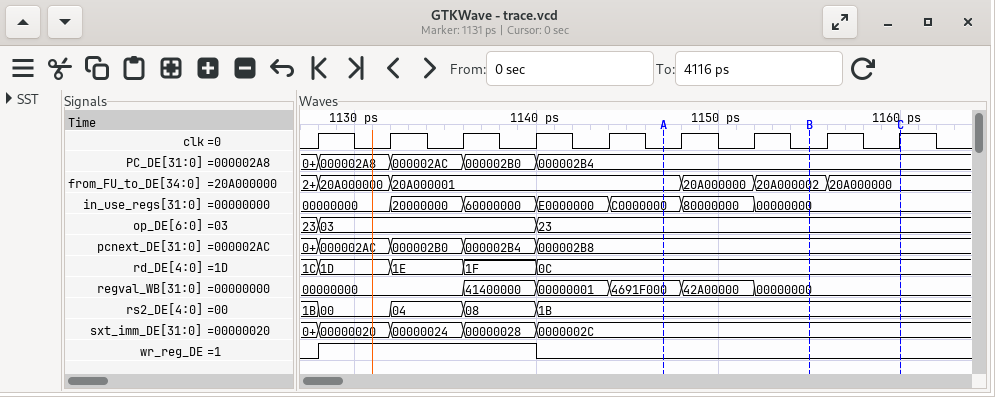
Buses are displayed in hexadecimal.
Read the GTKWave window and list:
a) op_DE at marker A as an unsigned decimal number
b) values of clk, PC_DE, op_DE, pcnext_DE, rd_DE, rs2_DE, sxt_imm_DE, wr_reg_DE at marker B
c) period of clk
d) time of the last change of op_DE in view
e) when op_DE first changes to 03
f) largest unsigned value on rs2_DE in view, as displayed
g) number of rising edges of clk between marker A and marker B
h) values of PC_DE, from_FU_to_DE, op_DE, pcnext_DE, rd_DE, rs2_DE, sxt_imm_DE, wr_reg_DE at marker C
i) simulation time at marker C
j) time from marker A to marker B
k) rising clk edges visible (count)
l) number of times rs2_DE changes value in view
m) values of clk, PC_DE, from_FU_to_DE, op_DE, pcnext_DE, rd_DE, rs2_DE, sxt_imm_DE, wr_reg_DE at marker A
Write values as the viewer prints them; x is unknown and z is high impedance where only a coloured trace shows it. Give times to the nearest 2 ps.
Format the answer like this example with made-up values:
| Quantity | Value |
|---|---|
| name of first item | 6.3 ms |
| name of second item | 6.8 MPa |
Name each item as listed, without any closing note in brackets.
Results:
| Quantity | Value |
|---|---|
| op_DE at marker A as an unsigned decimal number | 35 |
| values of clk, PC_DE, op_DE, pcnext_DE, rd_DE, rs2_DE, sxt_imm_DE, wr_reg_DE at marker B | clk=0, PC_DE=000002B4, op_DE=23, pcnext_DE=000002B8, rd_DE=0C, rs2_DE=1B, sxt_imm_DE=0000002C, wr_reg_DE=0 |
| period of clk | 4 ps |
| time of the last change of op_DE in view | 1140 ps |
| when op_DE first changes to 03 | 1128 ps |
| largest unsigned value on rs2_DE in view, as displayed | 1B |
| number of rising edges of clk between marker A and marker B | 2 |
| values of PC_DE, from_FU_to_DE, op_DE, pcnext_DE, rd_DE, rs2_DE, sxt_imm_DE, wr_reg_DE at marker C | PC_DE=000002B4, from_FU_to_DE=20A000000, op_DE=23, pcnext_DE=000002B8, rd_DE=0C, rs2_DE=1B, sxt_imm_DE=0000002C, wr_reg_DE=0 |
| simulation time at marker C | 1160 ps |
| time from marker A to marker B | 8 ps |
| rising clk edges visible | 9 |
| number of times rs2_DE changes value in view | 4 |
| values of clk, PC_DE, from_FU_to_DE, op_DE, pcnext_DE, rd_DE, rs2_DE, sxt_imm_DE, wr_reg_DE at marker A | clk=0, PC_DE=000002B4, from_FU_to_DE=20A000001, op_DE=23, pcnext_DE=000002B8, rd_DE=0C, rs2_DE=1B, sxt_imm_DE=0000002C, wr_reg_DE=0 |
